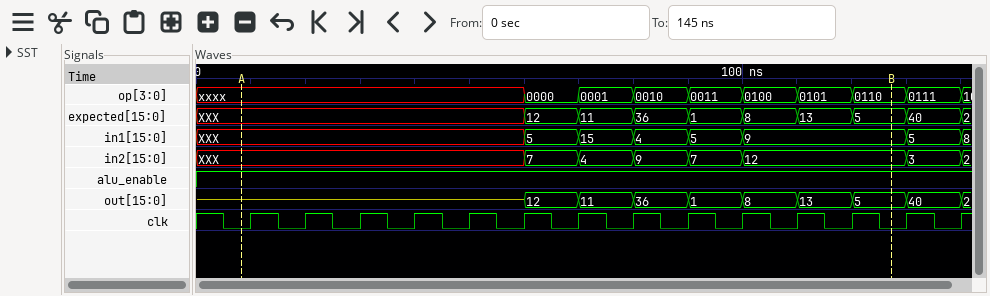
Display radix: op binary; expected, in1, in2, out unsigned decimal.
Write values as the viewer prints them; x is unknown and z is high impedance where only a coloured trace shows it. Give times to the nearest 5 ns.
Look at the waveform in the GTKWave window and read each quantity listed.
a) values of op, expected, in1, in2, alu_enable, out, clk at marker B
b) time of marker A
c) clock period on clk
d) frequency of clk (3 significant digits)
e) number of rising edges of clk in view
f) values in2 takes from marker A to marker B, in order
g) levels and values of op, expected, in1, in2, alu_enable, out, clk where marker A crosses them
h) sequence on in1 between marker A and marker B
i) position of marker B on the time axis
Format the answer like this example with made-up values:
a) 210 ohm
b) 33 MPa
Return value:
a) op=0110, expected=5, in1=9, in2=12, alu_enable=1, out=5, clk=0
b) 10 ns
c) 10 ns
d) 100 MHz
e) 14
f) XXX, 7, 4, 9, 7, 12
g) op=xxxx, expected=XXX, in1=XXX, in2=XXX, alu_enable=1, out=z, clk=0
h) XXX, 5, 15, 4, 5, 9
i) 125 ns
